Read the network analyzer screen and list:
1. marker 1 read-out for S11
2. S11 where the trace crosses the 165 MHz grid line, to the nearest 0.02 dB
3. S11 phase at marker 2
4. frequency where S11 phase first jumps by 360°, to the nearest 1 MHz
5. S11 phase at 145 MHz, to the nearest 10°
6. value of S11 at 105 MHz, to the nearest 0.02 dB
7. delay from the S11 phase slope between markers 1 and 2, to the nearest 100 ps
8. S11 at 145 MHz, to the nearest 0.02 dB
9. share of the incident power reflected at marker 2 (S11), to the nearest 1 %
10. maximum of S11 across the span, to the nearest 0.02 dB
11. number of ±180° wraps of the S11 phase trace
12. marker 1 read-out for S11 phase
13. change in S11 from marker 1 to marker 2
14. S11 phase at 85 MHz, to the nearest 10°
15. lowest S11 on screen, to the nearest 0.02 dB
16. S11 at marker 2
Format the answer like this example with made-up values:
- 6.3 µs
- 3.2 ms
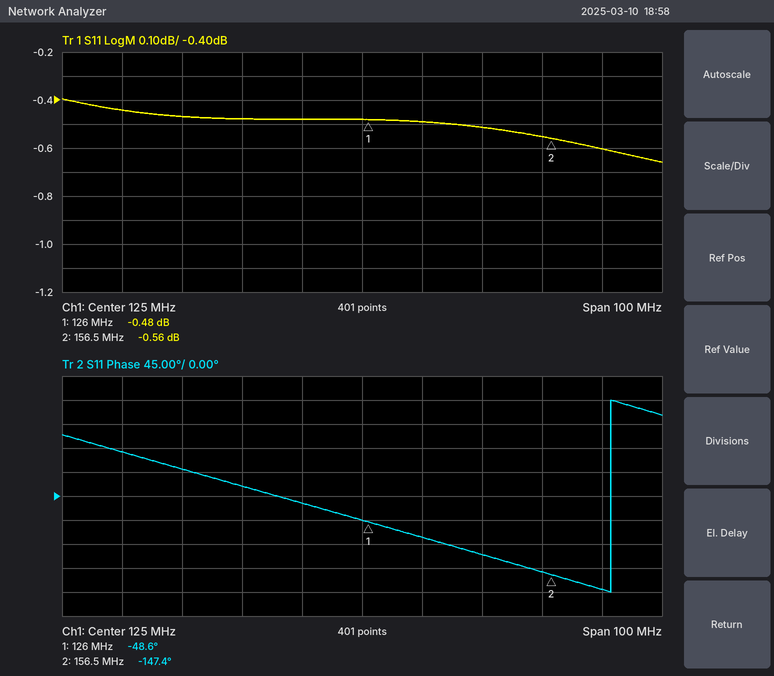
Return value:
- -0.48 dB
- -0.60 dB
- -147.4°
- 166 MHz
- -110°
- -0.48 dB
- 9.0 ns
- -0.52 dB
- 88 %
- -0.40 dB
- 1
- -48.6°
- -0.08 dB
- 80°
- -0.66 dB
- -0.56 dB
